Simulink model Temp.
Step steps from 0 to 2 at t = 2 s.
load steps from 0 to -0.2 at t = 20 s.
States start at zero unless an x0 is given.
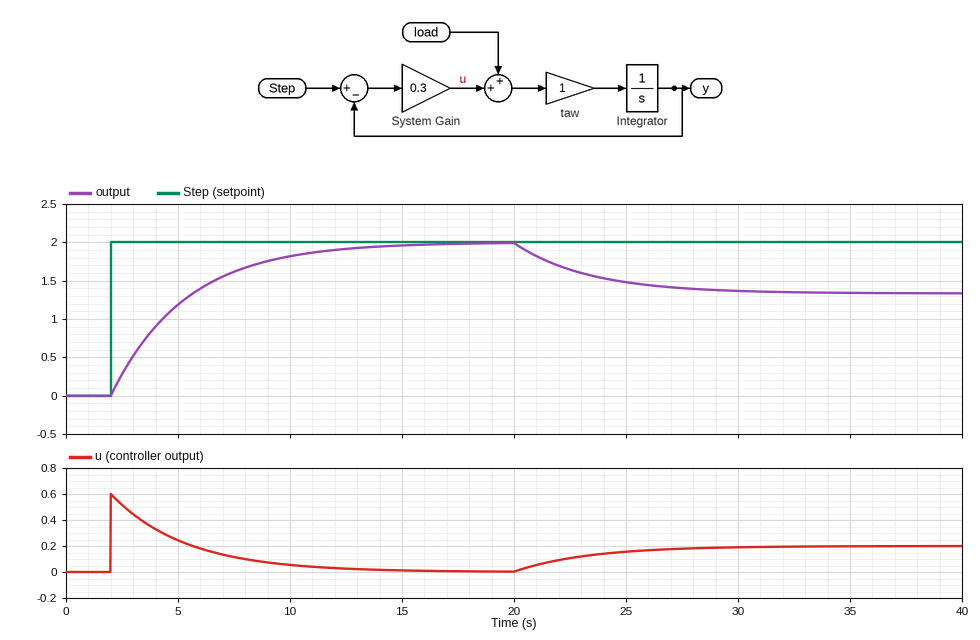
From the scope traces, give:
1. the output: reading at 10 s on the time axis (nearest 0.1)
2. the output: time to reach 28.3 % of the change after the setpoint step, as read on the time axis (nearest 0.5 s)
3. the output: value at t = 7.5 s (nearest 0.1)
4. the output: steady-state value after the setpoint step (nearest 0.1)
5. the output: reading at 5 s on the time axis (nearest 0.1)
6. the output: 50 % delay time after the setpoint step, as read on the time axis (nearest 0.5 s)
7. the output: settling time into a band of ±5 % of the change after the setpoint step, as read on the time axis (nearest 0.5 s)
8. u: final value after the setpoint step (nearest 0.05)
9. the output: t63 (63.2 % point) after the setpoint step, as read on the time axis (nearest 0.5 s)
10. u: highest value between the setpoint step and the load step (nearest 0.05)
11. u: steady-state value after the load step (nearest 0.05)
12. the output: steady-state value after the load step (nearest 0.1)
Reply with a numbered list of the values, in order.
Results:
1. 1.8
2. 3.0 s
3. 1.6
4. 2.0
5. 1.2
6. 4.5 s
7. 12.0 s
8. 0.00
9. 5.5 s
10. 0.60
11. 0.20
12. 1.3
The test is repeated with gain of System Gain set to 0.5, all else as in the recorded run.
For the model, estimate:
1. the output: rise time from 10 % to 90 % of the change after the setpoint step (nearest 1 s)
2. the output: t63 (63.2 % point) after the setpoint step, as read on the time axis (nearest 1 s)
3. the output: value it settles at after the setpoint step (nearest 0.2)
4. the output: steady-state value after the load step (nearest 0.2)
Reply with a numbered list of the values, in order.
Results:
1. 4 s
2. 4 s
3. 2.0
4. 1.6
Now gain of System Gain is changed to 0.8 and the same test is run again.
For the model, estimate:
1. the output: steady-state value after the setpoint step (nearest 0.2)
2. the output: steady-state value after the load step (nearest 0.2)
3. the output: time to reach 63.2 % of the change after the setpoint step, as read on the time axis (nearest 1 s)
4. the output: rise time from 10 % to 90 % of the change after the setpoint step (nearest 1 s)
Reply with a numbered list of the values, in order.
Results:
1. 2.0
2. 1.8
3. 3 s
4. 3 s
